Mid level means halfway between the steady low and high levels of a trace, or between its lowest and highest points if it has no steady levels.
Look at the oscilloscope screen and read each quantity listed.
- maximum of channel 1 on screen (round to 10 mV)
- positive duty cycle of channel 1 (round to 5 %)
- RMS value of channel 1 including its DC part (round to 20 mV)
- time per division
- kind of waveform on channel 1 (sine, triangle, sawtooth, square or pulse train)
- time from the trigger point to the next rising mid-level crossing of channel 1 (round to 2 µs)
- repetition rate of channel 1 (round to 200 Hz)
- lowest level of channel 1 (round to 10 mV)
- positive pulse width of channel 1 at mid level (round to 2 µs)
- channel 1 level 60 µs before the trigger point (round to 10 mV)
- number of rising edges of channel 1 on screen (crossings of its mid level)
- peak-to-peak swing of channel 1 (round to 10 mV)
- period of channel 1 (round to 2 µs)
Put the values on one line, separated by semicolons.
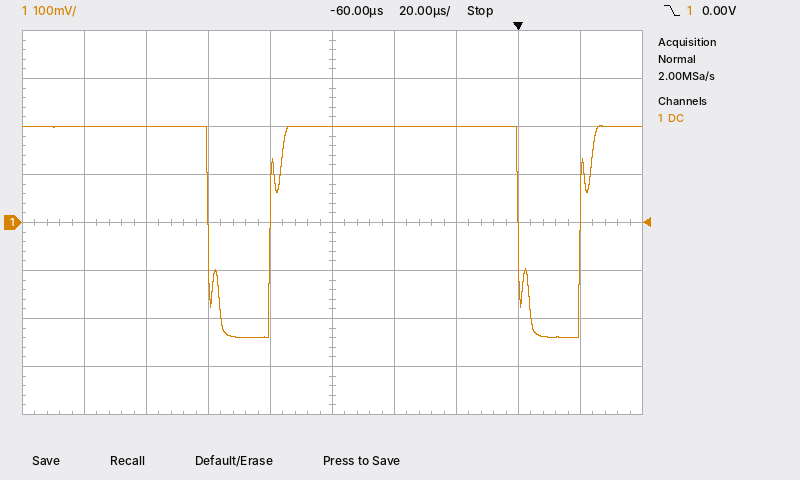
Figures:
200 mV; 80 %; 200 mV; 20 µs; pulse train; 20 µs; 10.0 kHz; -240 mV; 80 µs; 200 mV; 2; 440 mV; 100 µs
